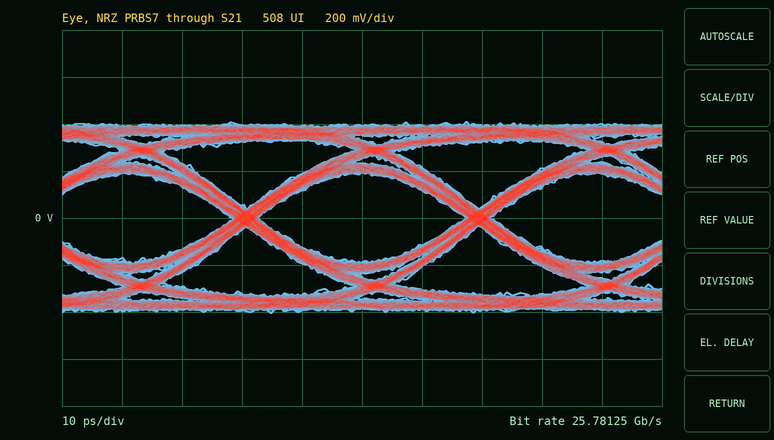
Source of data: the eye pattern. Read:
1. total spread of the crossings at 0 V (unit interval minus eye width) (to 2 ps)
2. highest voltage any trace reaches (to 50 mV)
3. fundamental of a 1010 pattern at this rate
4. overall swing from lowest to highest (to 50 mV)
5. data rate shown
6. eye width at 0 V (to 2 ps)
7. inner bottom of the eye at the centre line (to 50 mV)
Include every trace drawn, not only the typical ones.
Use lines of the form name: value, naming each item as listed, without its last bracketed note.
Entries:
total spread of the crossings at 0 V (unit interval minus eye width): 4 ps
highest voltage any trace reaches: 400 mV
fundamental of a 1010 pattern at this rate: 12.89062 GHz
overall swing from lowest to highest: 800 mV
data rate shown: 25.78125 Gb/s
eye width at 0 V: 34 ps
inner bottom of the eye at the centre line: -200 mV
